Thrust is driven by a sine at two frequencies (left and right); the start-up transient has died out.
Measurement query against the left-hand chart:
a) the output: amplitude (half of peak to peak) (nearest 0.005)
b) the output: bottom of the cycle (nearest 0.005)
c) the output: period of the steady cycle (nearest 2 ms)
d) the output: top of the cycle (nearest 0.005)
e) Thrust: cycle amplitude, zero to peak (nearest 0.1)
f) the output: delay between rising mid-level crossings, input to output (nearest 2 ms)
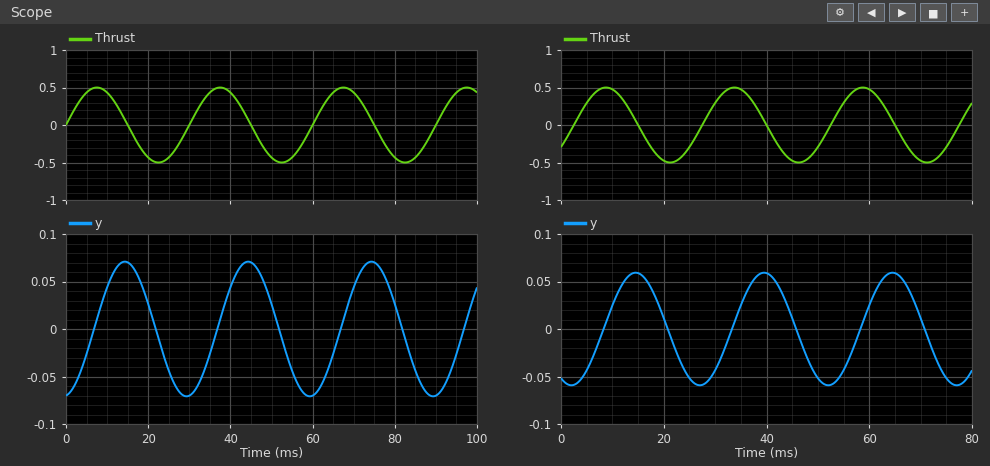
0.070
-0.070
30 ms
0.070
0.5
6 ms
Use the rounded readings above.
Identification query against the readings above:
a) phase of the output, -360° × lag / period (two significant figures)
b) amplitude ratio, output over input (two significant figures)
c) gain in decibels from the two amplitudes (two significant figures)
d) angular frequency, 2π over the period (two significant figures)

-72°
0.14
-17 dB
0.21 rad/ms
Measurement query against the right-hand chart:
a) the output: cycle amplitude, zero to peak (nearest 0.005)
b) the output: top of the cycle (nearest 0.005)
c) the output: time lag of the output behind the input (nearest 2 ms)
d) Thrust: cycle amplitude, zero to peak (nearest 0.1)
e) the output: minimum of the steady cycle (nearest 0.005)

0.060
0.060
6 ms
0.5
-0.060
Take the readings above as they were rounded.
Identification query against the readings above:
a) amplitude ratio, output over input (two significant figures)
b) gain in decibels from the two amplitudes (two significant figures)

0.12
-18 dB
